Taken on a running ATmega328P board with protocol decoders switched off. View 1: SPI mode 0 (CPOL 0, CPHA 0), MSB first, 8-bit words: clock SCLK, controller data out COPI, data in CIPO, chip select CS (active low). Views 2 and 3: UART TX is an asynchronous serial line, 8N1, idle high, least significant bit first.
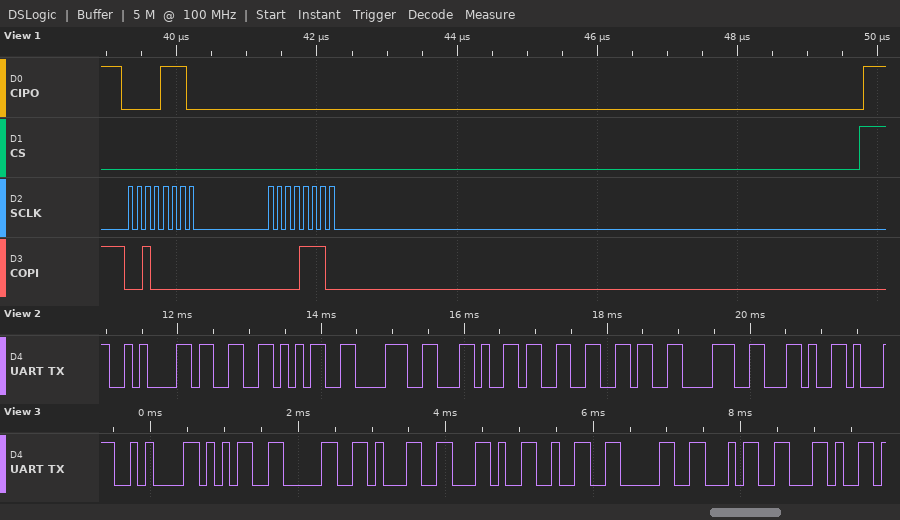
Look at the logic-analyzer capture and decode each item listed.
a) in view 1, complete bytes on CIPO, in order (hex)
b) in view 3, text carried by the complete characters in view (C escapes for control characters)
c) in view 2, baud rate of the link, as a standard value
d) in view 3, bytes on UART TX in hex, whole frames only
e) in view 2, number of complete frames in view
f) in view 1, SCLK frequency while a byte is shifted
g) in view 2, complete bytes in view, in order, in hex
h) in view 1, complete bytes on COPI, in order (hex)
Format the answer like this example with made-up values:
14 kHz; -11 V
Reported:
0E 00; "\n501,204,"; 9600 baud; 0A 35 30 31 2C 32 30 34 2C; 9; 8 MHz; 0A 33 35 38 2C 33 36 38 2C; 20 0E
